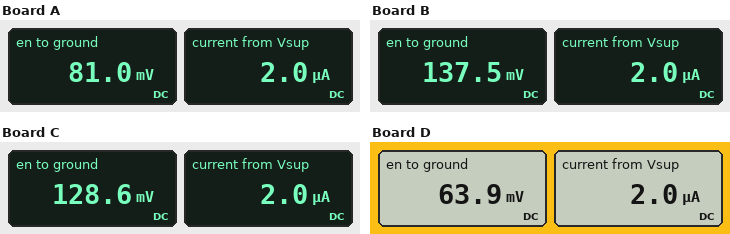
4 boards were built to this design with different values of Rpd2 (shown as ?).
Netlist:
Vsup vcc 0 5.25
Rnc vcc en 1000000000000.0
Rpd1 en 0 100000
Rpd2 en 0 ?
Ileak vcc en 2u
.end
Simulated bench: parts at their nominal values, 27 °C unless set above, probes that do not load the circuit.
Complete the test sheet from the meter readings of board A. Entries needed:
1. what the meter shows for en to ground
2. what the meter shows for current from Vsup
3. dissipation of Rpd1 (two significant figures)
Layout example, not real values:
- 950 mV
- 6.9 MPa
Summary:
- 81.0 mV
- 2.0 µA
- 66 nW
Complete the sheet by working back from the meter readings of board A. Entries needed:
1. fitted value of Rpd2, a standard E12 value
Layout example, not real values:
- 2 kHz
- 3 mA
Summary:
- 68 kΩ
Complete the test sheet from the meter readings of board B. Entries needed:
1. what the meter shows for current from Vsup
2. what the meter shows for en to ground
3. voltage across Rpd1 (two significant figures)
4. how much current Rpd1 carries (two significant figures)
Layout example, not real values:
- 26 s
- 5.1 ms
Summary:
- 2.0 µA
- 137.5 mV
- 140 mV
- 1.4 µA
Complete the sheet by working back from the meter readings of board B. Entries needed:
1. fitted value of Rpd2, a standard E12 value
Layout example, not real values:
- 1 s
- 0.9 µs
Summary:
- 220 kΩ
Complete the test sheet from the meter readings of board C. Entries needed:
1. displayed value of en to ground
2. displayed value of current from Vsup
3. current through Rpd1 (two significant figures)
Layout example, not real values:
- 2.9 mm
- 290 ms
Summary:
- 128.6 mV
- 2.0 µA
- 1.3 µA
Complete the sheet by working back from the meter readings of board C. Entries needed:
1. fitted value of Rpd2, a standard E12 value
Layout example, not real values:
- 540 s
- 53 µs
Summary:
- 180 kΩ
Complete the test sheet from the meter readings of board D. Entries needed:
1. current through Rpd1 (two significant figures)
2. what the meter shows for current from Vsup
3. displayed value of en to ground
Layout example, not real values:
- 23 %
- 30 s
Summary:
- 640 nA
- 2.0 µA
- 63.9 mV
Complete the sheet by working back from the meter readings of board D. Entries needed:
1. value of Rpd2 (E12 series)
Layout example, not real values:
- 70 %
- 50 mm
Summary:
- 47 kΩ
